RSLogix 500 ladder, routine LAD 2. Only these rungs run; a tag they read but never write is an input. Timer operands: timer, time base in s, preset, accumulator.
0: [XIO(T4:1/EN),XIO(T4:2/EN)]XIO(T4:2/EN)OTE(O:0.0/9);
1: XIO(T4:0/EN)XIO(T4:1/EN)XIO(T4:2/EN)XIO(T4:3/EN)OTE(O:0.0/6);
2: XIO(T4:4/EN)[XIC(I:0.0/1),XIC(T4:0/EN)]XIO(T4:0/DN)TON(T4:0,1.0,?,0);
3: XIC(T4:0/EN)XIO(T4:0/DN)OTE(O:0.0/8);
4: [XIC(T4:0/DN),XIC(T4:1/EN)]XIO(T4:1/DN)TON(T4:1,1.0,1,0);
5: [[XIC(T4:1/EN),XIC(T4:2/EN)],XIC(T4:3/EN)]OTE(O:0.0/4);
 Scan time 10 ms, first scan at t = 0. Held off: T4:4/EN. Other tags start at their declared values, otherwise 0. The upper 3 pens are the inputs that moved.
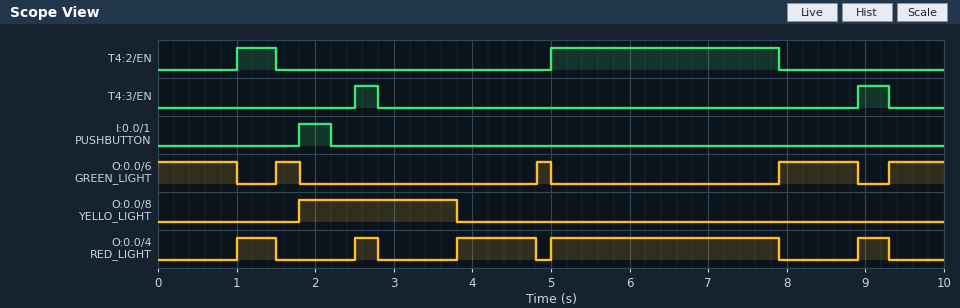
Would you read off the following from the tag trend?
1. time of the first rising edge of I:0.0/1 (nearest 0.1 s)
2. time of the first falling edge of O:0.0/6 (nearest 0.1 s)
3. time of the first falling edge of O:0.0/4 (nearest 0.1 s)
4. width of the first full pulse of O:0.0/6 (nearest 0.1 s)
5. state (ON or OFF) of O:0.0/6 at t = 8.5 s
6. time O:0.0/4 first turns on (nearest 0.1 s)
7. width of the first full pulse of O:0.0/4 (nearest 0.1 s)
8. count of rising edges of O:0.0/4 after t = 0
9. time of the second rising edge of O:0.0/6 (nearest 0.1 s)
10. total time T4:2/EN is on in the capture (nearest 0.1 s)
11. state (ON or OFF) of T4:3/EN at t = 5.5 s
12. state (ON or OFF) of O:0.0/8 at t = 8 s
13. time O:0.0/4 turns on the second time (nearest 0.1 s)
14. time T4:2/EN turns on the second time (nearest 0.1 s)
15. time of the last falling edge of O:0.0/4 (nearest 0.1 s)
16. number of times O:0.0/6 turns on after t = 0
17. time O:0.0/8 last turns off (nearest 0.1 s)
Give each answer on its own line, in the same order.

1.8 s
1.0 s
1.5 s
0.3 s
ON
1.0 s
0.5 s
5
4.8 s
3.4 s
OFF
OFF
2.5 s
5.0 s
9.3 s
4
3.8 s
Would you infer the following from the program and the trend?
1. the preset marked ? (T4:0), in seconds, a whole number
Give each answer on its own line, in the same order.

2 s
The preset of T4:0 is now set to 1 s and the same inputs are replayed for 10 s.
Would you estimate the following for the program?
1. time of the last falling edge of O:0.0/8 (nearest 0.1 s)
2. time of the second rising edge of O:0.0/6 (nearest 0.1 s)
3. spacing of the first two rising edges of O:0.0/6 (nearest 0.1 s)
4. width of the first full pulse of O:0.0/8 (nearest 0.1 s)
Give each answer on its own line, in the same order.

2.8 s
3.8 s
2.3 s
1.0 s
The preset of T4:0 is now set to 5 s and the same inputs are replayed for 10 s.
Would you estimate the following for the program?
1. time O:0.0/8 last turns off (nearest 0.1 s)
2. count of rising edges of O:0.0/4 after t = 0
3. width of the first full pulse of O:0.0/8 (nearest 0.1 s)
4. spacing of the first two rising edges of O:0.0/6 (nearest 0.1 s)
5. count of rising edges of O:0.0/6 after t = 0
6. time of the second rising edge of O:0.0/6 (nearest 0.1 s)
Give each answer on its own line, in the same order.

6.8 s
4
5.0 s
6.4 s
3
7.9 s
